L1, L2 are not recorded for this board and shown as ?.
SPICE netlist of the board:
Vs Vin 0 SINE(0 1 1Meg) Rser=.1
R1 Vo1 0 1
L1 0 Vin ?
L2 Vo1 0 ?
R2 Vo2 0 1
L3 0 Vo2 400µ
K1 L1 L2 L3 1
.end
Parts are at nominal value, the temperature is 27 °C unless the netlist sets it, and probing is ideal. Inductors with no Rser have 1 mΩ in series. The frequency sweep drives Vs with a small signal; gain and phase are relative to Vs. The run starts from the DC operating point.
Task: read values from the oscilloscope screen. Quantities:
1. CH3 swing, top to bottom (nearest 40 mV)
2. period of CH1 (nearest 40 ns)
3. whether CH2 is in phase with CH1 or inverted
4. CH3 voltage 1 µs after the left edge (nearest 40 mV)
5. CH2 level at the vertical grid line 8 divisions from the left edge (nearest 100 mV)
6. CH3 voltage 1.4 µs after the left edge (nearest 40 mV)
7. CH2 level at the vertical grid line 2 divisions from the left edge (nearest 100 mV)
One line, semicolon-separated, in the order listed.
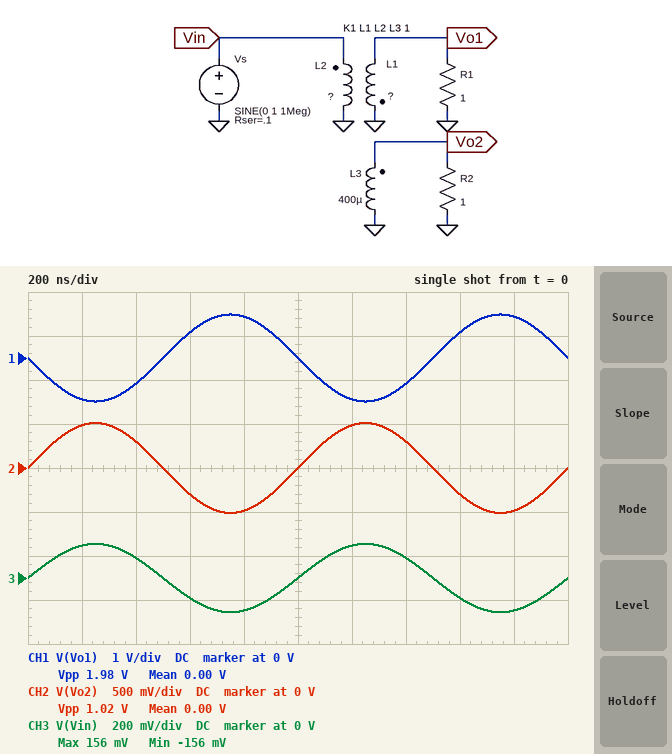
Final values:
320 mV; 1.00 µs; inverted; 0 V; -300 mV; 80 mV; 300 mV
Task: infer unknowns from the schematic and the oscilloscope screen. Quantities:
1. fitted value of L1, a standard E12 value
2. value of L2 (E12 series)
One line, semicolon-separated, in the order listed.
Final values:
33 µH; 1.5 mH
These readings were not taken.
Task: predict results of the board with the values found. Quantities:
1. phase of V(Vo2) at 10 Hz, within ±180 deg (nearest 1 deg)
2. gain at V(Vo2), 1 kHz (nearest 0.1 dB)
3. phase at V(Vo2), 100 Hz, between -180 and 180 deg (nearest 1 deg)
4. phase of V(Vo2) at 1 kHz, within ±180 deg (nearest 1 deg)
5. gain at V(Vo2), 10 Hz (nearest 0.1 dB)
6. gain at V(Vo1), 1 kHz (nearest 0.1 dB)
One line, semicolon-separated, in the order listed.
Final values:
82 deg; -5.9 dB; 36 deg; 4 deg; -23.0 dB; -0.1 dB
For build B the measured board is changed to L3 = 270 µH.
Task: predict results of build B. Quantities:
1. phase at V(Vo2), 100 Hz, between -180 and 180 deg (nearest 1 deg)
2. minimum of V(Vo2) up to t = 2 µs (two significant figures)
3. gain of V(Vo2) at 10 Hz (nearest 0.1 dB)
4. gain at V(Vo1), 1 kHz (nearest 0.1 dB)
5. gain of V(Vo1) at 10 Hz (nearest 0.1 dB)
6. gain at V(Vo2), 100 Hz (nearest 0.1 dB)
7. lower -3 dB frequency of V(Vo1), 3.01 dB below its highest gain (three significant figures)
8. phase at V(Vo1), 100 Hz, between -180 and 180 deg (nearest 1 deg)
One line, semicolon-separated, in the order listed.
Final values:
37 deg; -450 mV; -24.7 dB; 0.4 dB; -17.3 dB; -9.0 dB; 76.0 Hz; -143 deg
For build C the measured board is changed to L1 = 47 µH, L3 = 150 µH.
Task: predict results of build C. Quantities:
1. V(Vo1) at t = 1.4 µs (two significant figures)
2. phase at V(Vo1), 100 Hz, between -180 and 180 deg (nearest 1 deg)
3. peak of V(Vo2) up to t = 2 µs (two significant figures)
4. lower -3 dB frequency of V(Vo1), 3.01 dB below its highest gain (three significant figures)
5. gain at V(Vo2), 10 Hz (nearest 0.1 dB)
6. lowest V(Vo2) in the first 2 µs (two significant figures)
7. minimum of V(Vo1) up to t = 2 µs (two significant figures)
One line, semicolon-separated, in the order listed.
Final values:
-730 mV; -143 deg; 390 mV; 75.3 Hz; -25.7 dB; -390 mV; -1.2 V
